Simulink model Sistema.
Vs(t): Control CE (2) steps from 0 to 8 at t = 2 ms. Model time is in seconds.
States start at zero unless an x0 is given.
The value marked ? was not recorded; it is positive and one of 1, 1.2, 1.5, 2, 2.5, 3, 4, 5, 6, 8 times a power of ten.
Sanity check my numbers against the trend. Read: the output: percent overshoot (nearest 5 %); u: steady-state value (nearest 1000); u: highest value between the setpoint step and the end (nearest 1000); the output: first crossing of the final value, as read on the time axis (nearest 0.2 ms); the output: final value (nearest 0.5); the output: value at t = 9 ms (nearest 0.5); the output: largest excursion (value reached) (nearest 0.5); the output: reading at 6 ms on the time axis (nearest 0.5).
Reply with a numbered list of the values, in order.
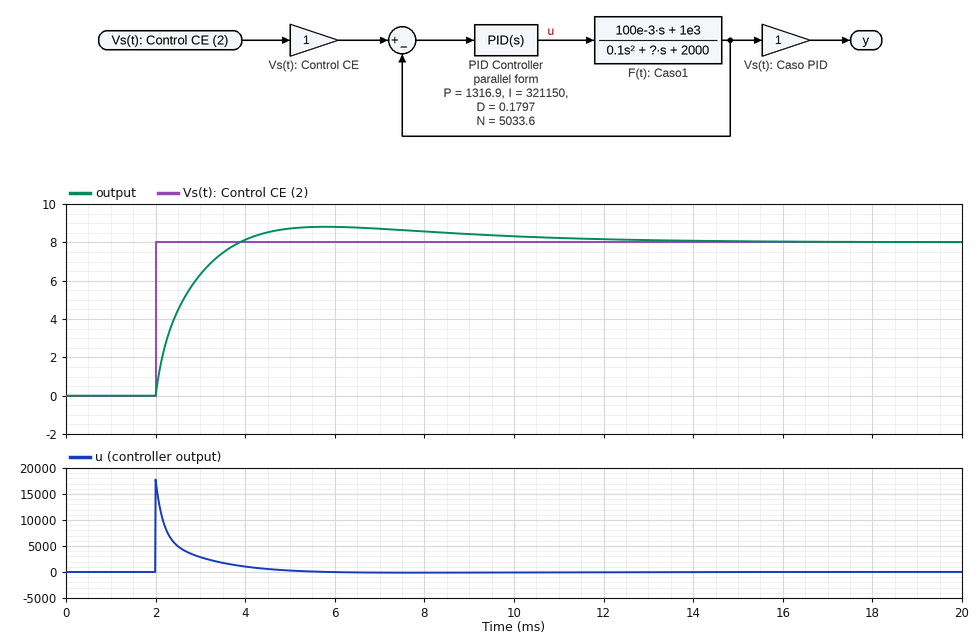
1. 10 %
2. 0
3. 18000
4. 3.8 ms
5. 8.0
6. 8.5
7. 9.0
8. 9.0
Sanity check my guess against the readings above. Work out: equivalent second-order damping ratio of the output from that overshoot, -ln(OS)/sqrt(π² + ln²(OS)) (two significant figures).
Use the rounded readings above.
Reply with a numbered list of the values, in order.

1. 0.59
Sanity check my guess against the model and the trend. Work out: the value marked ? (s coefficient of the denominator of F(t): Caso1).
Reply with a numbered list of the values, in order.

1. 1000
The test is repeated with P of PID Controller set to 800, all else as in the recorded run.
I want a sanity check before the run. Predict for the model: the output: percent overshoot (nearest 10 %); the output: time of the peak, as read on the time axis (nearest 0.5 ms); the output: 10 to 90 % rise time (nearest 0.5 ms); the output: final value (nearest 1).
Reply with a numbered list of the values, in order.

1. 20 %
2. 6.5 ms
3. 1.5 ms
4. 8
